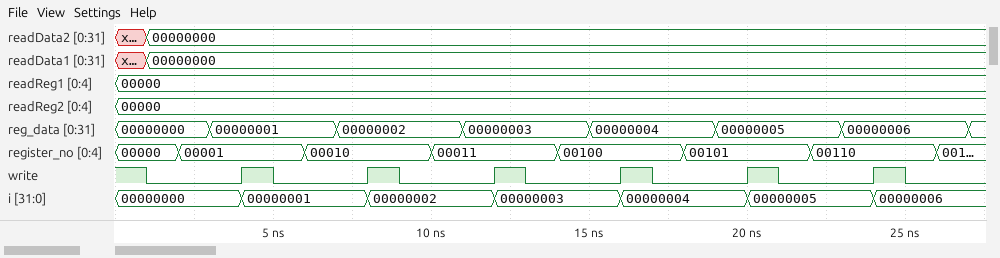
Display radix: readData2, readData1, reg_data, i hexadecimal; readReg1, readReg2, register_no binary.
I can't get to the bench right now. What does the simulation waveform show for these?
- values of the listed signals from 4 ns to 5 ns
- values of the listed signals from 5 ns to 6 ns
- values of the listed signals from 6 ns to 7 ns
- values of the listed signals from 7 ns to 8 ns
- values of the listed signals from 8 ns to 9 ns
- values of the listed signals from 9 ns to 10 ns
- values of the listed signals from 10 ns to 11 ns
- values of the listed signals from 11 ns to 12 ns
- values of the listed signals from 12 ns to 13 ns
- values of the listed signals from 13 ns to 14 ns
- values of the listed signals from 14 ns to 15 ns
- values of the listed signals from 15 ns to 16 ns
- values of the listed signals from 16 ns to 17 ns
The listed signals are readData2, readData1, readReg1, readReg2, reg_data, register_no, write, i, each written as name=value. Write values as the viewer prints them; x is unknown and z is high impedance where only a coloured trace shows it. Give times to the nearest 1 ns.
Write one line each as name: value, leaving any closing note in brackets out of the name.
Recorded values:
values of the listed signals from 4 ns to 5 ns: readData2=00000000, readData1=00000000, readReg1=00000, readReg2=00000, reg_data=00000001, register_no=00001, write=1, i=00000001
values of the listed signals from 5 ns to 6 ns: readData2=00000000, readData1=00000000, readReg1=00000, readReg2=00000, reg_data=00000001, register_no=00001, write=0, i=00000001
values of the listed signals from 6 ns to 7 ns: readData2=00000000, readData1=00000000, readReg1=00000, readReg2=00000, reg_data=00000001, register_no=00010, write=0, i=00000001
values of the listed signals from 7 ns to 8 ns: readData2=00000000, readData1=00000000, readReg1=00000, readReg2=00000, reg_data=00000002, register_no=00010, write=0, i=00000001
values of the listed signals from 8 ns to 9 ns: readData2=00000000, readData1=00000000, readReg1=00000, readReg2=00000, reg_data=00000002, register_no=00010, write=1, i=00000002
values of the listed signals from 9 ns to 10 ns: readData2=00000000, readData1=00000000, readReg1=00000, readReg2=00000, reg_data=00000002, register_no=00010, write=0, i=00000002
values of the listed signals from 10 ns to 11 ns: readData2=00000000, readData1=00000000, readReg1=00000, readReg2=00000, reg_data=00000002, register_no=00011, write=0, i=00000002
values of the listed signals from 11 ns to 12 ns: readData2=00000000, readData1=00000000, readReg1=00000, readReg2=00000, reg_data=00000003, register_no=00011, write=0, i=00000002
values of the listed signals from 12 ns to 13 ns: readData2=00000000, readData1=00000000, readReg1=00000, readReg2=00000, reg_data=00000003, register_no=00011, write=1, i=00000003
values of the listed signals from 13 ns to 14 ns: readData2=00000000, readData1=00000000, readReg1=00000, readReg2=00000, reg_data=00000003, register_no=00011, write=0, i=00000003
values of the listed signals from 14 ns to 15 ns: readData2=00000000, readData1=00000000, readReg1=00000, readReg2=00000, reg_data=00000003, register_no=00100, write=0, i=00000003
values of the listed signals from 15 ns to 16 ns: readData2=00000000, readData1=00000000, readReg1=00000, readReg2=00000, reg_data=00000004, register_no=00100, write=0, i=00000003
values of the listed signals from 16 ns to 17 ns: readData2=00000000, readData1=00000000, readReg1=00000, readReg2=00000, reg_data=00000004, register_no=00100, write=1, i=00000004
